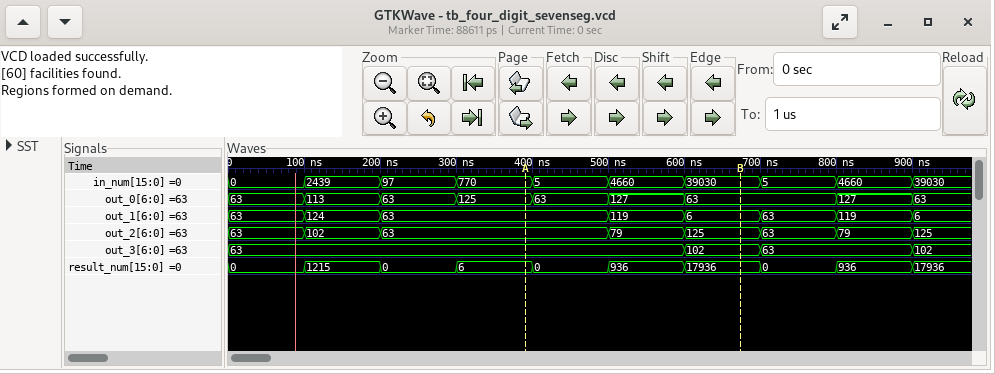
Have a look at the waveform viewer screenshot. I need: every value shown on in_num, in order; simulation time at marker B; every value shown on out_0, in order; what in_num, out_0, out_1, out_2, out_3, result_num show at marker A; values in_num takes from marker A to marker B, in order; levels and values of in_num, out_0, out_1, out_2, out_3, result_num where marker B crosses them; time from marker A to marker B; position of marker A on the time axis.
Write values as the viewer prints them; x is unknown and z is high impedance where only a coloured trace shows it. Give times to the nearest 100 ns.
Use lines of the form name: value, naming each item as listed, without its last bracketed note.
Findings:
every value shown on in_num, in order: 0, 2439, 97, 770, 5, 4660, 39030, 5, 4660, 39030
simulation time at marker B: 700 ns
every value shown on out_0, in order: 63, 113, 63, 125, 63, 127, 63, 127, 63
what in_num, out_0, out_1, out_2, out_3, result_num show at marker A: in_num=770, out_0=125, out_1=63, out_2=63, out_3=63, result_num=6
values in_num takes from marker A to marker B, in order: 770, 5, 4660, 39030
levels and values of in_num, out_0, out_1, out_2, out_3, result_num where marker B crosses them: in_num=39030, out_0=63, out_1=6, out_2=125, out_3=102, result_num=17936
time from marker A to marker B: 300 ns
position of marker A on the time axis: 400 ns
